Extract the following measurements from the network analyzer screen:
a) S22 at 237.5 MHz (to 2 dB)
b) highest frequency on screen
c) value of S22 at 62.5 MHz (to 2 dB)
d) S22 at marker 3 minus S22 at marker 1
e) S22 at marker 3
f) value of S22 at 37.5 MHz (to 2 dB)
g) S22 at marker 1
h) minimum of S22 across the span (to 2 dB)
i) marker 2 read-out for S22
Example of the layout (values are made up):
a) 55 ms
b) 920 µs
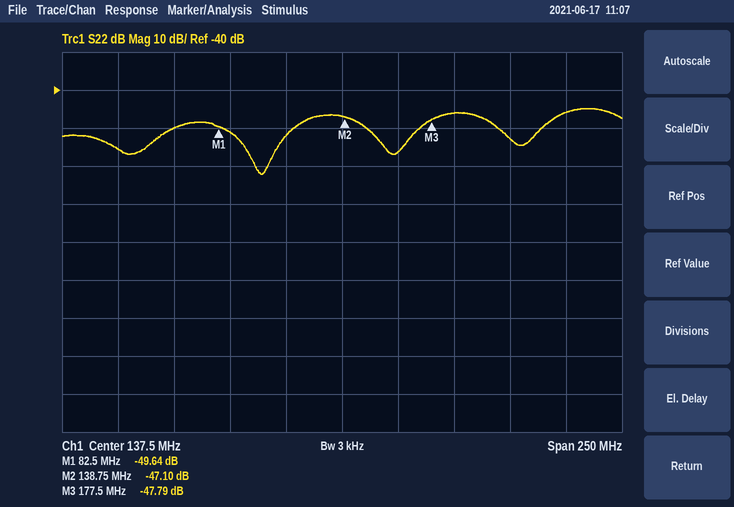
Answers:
a) -46 dB
b) 262.5 MHz
c) -50 dB
d) 1.85 dB
e) -47.79 dB
f) -56 dB
g) -49.64 dB
h) -62 dB
i) -47.10 dB
